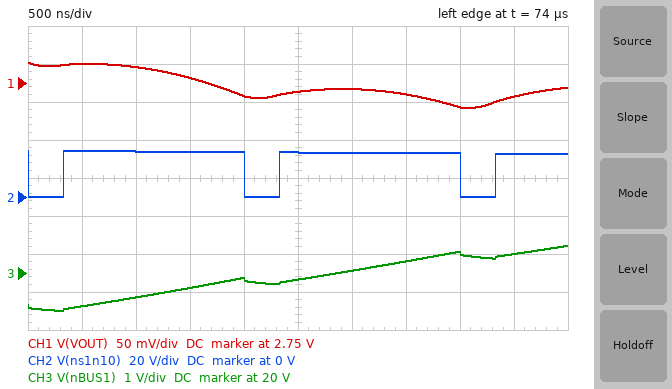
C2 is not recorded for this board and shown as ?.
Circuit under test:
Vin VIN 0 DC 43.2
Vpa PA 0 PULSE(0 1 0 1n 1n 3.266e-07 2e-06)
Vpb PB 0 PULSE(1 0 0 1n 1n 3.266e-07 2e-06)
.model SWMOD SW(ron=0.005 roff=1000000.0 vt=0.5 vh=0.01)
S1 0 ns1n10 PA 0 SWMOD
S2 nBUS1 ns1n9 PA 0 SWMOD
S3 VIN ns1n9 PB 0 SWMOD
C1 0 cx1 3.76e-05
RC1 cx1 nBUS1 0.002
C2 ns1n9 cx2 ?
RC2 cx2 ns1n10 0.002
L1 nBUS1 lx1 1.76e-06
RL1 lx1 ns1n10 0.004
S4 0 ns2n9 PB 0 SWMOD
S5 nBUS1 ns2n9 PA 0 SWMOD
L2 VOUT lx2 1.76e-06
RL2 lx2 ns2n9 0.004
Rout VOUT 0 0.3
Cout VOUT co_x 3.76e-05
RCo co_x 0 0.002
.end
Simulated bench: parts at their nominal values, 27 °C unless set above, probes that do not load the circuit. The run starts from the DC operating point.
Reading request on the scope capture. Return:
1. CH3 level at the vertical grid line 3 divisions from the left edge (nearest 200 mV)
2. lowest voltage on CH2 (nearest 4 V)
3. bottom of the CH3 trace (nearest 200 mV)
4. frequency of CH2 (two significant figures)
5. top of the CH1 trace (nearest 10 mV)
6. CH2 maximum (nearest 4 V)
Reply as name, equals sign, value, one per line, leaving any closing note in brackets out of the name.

CH3 level at the vertical grid line 3 divisions from the left edge = 19.6 V
lowest voltage on CH2 = 0 V
bottom of the CH3 trace = 19.0 V
frequency of CH2 = 500 kHz
top of the CH1 trace = 2.78 V
CH2 maximum = 24 V
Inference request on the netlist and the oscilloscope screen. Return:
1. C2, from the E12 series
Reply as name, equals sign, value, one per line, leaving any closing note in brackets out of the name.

C2, from the E12 series = 56 µF
